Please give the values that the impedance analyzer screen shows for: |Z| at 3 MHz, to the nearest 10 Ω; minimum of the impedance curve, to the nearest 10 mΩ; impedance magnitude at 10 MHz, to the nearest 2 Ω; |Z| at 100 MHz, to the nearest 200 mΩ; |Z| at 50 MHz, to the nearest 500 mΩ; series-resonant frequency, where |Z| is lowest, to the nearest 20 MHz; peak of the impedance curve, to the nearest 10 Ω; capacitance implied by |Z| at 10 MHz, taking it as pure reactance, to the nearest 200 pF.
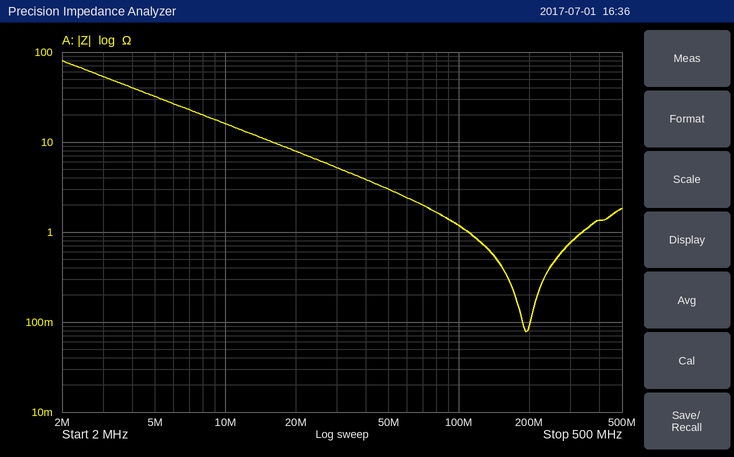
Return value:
50 Ω
80 mΩ
16 Ω
1.2 Ω
3.0 Ω
200 MHz
80 Ω
1.0 nF
